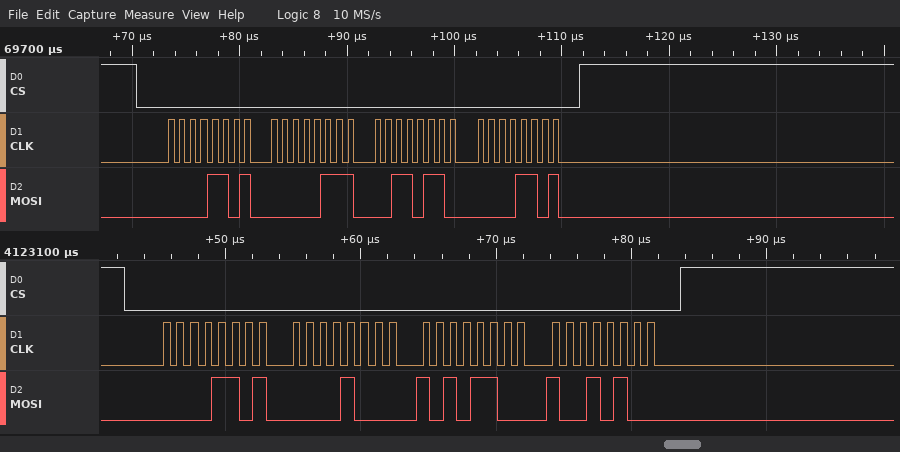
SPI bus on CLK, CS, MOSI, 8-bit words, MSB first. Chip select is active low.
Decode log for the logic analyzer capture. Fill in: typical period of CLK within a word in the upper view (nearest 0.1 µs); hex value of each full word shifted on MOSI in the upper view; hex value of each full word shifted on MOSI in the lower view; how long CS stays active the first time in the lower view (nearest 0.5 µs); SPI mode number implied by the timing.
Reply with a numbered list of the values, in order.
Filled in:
1. 1 µs
2. 0D, 07, 36, 0D
3. 0D, 08, AC, 94
4. 41 µs
5. 0
